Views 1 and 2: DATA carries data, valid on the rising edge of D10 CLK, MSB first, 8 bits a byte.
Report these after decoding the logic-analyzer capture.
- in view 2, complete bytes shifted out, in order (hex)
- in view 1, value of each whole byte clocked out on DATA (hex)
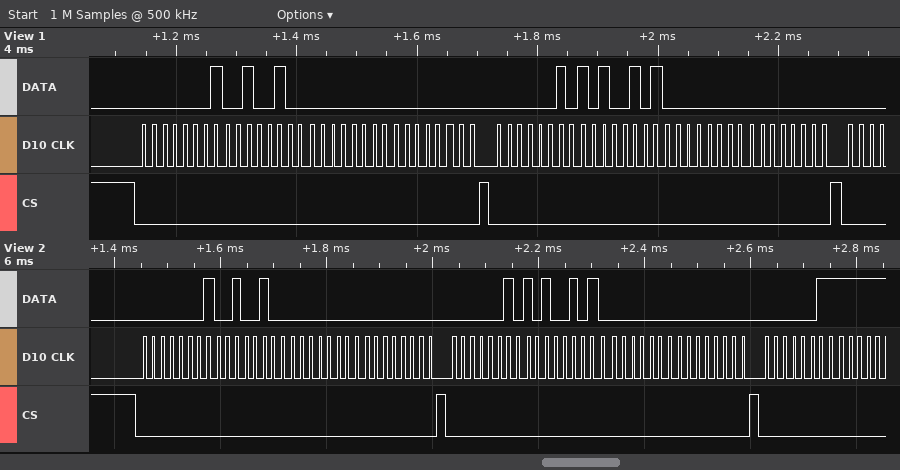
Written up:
01 24 00 00 02 A5 00 00 03
0x01 0x24 0x00 0x00 0x02 0xA5 0x00 0x00
